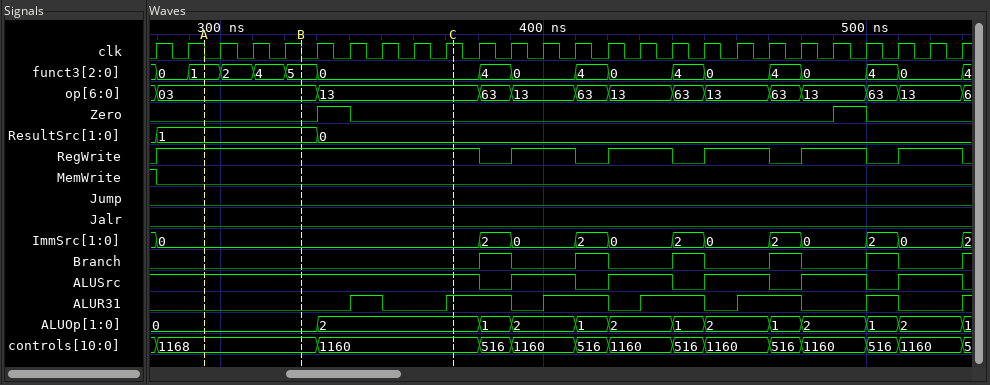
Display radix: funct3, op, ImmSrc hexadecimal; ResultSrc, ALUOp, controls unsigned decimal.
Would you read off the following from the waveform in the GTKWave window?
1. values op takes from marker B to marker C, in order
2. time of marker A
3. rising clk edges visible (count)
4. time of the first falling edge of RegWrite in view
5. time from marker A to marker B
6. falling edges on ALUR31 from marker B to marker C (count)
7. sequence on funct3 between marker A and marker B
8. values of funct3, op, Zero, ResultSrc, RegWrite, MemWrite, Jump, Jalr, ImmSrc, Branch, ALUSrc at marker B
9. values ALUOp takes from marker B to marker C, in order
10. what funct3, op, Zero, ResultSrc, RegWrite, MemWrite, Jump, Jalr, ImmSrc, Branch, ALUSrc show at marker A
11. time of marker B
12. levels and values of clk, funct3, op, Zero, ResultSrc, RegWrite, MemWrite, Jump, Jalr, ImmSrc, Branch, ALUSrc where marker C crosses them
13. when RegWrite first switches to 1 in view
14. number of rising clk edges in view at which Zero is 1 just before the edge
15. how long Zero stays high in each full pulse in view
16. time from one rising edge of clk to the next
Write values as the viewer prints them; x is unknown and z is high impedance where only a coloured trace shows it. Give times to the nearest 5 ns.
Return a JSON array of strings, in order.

["03, 13", "295 ns", "26", "380 ns", "30 ns", "1", "1, 2, 4, 5", "funct3=5, op=03, Zero=0, ResultSrc=1, RegWrite=1, MemWrite=0, Jump=0, Jalr=0, ImmSrc=0, Branch=0, ALUSrc=1", "0, 2", "funct3=1, op=03, Zero=0, ResultSrc=1, RegWrite=1, MemWrite=0, Jump=0, Jalr=0, ImmSrc=0, Branch=0, ALUSrc=1", "325 ns", "clk=1, funct3=0, op=13, Zero=0, ResultSrc=0, RegWrite=1, MemWrite=0, Jump=0, Jalr=0, ImmSrc=0, Branch=0, ALUSrc=1", "280 ns", "2", "10 ns, 10 ns", "10 ns"]
